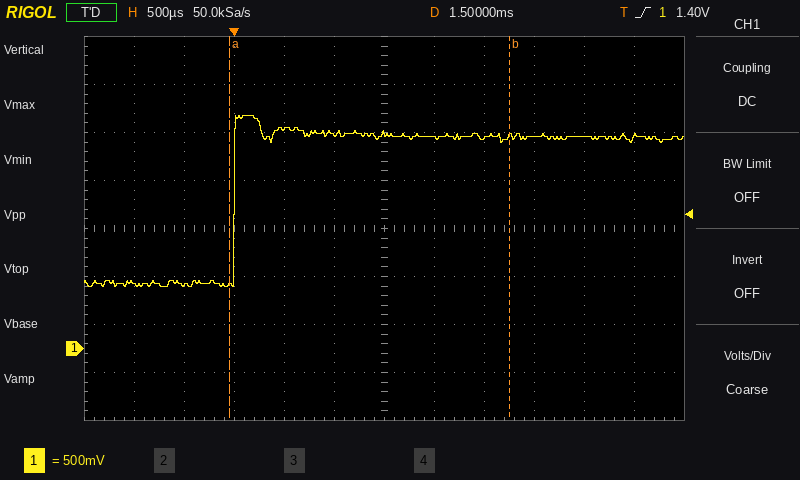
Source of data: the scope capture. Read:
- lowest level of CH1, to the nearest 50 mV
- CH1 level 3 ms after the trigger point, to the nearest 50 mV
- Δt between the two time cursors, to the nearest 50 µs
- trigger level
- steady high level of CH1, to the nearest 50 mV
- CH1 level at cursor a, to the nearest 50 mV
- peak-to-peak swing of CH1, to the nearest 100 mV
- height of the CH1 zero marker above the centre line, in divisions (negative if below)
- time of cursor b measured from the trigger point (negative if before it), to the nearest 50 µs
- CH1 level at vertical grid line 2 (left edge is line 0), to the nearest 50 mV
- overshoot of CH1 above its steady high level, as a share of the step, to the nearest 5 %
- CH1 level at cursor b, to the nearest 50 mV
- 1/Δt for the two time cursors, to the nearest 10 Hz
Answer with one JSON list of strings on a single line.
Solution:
["650 mV", "2.20 V", "2.80 ms", "1.40 V", "2.20 V", "650 mV", "1.80 V", "-2.5 div", "+2.75 ms", "650 mV", "15 %", "2.20 V", "360 Hz"]
